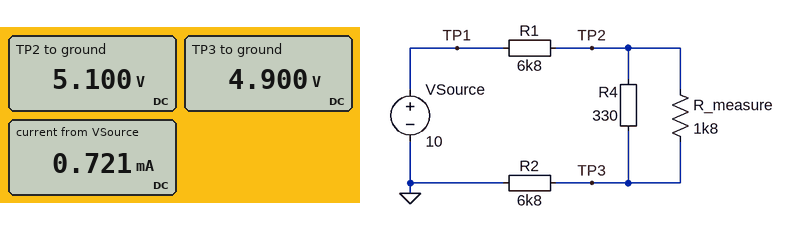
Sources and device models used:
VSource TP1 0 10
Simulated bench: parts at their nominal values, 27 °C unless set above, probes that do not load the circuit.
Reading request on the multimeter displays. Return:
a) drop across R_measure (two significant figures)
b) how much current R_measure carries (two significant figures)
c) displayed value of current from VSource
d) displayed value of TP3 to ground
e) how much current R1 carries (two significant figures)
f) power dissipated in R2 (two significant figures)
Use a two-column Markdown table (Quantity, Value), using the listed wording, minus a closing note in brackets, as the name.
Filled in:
| Quantity | Value |
|---|---|
| drop across R_measure | 200 mV |
| how much current R_measure carries | 110 µA |
| displayed value of current from VSource | 0.721 mA |
| displayed value of TP3 to ground | 4.900 V |
| how much current R1 carries | 720 µA |
| power dissipated in R2 | 3.5 mW |
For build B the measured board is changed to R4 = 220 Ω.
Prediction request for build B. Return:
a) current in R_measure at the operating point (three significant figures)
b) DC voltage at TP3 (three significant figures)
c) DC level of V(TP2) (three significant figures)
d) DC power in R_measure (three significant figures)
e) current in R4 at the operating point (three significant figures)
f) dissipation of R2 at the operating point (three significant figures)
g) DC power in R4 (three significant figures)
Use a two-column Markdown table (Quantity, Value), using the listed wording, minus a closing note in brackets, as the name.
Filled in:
| Quantity | Value |
|---|---|
| current in R_measure at the operating point | 78.9 µA |
| DC voltage at TP3 | 4.93 V |
| DC level of V(TP2) | 5.07 V |
| DC power in R_measure | 11.2 µW |
| current in R4 at the operating point | 646 µA |
| dissipation of R2 at the operating point | 3.57 mW |
| DC power in R4 | 91.8 µW |
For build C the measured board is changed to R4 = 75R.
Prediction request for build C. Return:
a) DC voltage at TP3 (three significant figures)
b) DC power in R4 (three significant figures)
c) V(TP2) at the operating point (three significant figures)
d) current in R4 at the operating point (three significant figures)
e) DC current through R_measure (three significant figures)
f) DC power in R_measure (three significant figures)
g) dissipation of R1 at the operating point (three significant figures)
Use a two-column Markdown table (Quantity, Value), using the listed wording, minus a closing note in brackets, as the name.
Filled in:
| Quantity | Value |
|---|---|
| DC voltage at TP3 | 4.97 V |
| DC power in R4 | 37.0 µW |
| V(TP2) at the operating point | 5.03 V |
| current in R4 at the operating point | 702 µA |
| DC current through R_measure | 29.3 µA |
| DC power in R_measure | 1.54 µW |
| dissipation of R1 at the operating point | 3.64 mW |
